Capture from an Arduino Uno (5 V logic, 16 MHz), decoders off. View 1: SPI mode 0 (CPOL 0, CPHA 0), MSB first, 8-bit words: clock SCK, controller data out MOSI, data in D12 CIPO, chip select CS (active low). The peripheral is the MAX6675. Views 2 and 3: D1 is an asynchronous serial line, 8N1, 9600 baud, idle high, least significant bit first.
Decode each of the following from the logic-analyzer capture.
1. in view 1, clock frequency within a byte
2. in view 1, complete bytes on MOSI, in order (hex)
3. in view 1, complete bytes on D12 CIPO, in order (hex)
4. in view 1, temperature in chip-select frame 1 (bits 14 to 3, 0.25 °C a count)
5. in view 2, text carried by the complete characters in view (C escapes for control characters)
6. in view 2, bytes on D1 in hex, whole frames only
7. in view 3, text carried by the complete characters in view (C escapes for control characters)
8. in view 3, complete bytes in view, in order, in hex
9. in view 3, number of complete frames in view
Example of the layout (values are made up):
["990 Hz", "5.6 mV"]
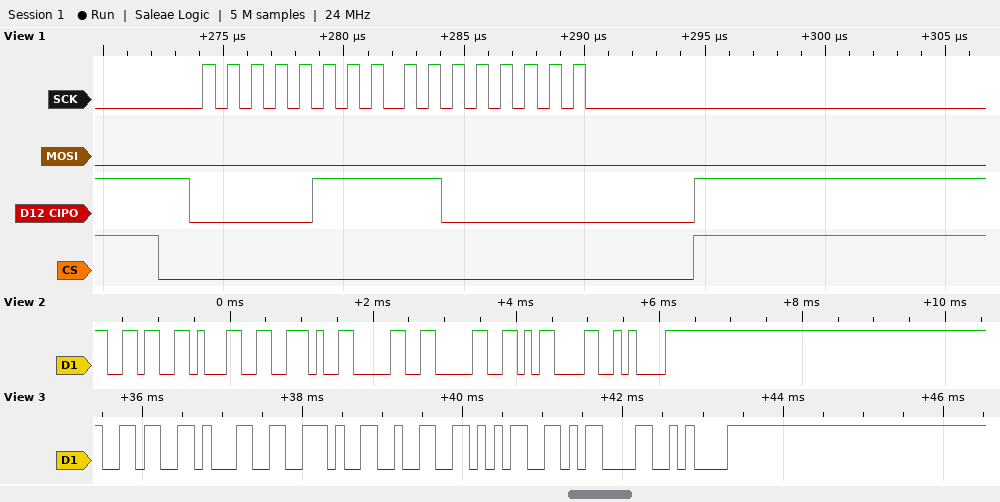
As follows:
["1 MHz", "0x00 0x00", "0x07 0xC0", "62.00 °C", "\"61.00\\r\\n\"", "0x36 0x31 0x2E 0x30 0x30 0x0D 0x0A", "\"61.25\\r\\n\"", "36 31 2E 32 35 0D 0A", "7"]
